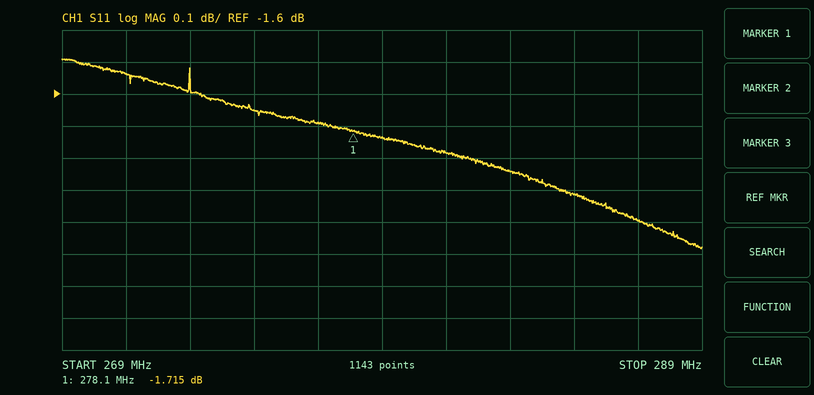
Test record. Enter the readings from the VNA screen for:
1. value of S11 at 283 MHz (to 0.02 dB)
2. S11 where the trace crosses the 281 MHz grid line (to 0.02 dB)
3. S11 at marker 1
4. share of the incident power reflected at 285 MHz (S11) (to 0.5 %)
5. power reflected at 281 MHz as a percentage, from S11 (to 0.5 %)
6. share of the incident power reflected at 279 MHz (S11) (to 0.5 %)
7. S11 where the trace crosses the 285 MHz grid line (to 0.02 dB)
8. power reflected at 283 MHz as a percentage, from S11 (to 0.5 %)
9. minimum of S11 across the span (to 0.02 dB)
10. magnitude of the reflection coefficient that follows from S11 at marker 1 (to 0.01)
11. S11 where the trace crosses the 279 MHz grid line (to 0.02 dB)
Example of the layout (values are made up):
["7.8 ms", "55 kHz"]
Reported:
["-1.84 dB", "-1.78 dB", "-1.715 dB", "64.5 %", "66.5 %", "67.0 %", "-1.92 dB", "65.5 %", "-2.08 dB", "0.82", "-1.74 dB"]
